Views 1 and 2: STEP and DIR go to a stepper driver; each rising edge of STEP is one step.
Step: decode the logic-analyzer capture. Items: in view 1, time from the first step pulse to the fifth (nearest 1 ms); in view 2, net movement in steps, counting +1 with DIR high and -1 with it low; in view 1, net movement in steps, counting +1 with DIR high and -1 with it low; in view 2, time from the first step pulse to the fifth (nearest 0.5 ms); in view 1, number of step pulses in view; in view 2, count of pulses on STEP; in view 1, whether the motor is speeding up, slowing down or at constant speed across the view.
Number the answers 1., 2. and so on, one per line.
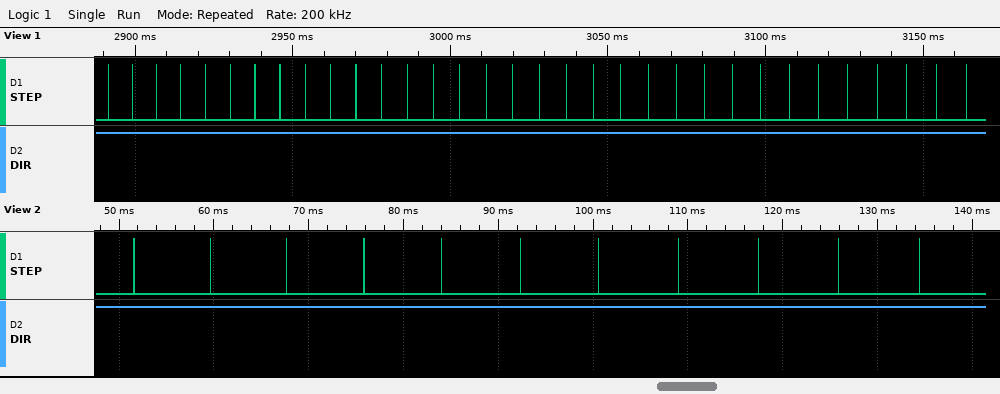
1. 31 ms
2. +11
3. +33
4. 32.5 ms
5. 33
6. 11
7. slowing down
